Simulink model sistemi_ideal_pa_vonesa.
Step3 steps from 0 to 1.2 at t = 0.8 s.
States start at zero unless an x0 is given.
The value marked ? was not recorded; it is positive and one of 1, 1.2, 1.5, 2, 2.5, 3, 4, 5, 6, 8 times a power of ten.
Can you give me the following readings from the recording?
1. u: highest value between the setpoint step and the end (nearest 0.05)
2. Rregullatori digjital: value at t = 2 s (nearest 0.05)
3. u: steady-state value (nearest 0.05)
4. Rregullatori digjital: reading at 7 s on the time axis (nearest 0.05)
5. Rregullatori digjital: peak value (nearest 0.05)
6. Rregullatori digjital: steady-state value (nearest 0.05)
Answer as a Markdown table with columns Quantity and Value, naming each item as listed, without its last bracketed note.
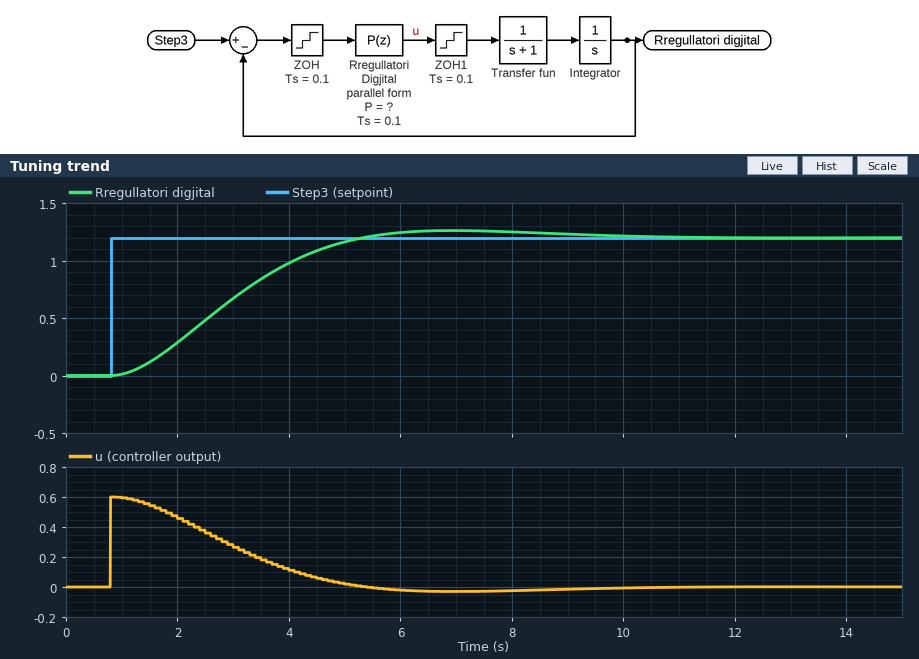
| Quantity | Value |
|---|---|
| u: highest value between the setpoint step and the end | 0.60 |
| Rregullatori digjital: value at t = 2 s | 0.30 |
| u: steady-state value | 0.00 |
| Rregullatori digjital: reading at 7 s on the time axis | 1.25 |
| Rregullatori digjital: peak value | 1.25 |
| Rregullatori digjital: steady-state value | 1.20 |
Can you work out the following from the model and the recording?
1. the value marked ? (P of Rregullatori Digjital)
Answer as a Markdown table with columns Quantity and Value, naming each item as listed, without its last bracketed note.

| Quantity | Value |
|---|---|
| the value marked ? | 0.5 |
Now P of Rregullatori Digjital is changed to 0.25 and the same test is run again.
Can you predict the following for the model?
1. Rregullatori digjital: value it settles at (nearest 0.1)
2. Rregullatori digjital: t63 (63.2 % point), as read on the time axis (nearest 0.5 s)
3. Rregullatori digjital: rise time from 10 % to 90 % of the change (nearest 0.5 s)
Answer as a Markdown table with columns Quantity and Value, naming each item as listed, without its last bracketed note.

| Quantity | Value |
|---|---|
| Rregullatori digjital: value it settles at | 1.2 |
| Rregullatori digjital: t63 (63.2 % point), as read on the time axis | 5.0 s |
| Rregullatori digjital: rise time from 10 % to 90 % of the change | 6.5 s |
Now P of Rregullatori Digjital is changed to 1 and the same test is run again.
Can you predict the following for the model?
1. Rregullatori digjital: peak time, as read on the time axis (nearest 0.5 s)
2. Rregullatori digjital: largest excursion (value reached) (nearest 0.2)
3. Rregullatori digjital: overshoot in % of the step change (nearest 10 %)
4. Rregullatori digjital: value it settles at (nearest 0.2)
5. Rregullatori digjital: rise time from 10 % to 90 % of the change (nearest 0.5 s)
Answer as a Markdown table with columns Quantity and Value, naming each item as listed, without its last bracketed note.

| Quantity | Value |
|---|---|
| Rregullatori digjital: peak time, as read on the time axis | 4.5 s |
| Rregullatori digjital: largest excursion (value reached) | 1.4 |
| Rregullatori digjital: overshoot in % of the step change | 20 % |
| Rregullatori digjital: value it settles at | 1.2 |
| Rregullatori digjital: rise time from 10 % to 90 % of the change | 1.5 s |
